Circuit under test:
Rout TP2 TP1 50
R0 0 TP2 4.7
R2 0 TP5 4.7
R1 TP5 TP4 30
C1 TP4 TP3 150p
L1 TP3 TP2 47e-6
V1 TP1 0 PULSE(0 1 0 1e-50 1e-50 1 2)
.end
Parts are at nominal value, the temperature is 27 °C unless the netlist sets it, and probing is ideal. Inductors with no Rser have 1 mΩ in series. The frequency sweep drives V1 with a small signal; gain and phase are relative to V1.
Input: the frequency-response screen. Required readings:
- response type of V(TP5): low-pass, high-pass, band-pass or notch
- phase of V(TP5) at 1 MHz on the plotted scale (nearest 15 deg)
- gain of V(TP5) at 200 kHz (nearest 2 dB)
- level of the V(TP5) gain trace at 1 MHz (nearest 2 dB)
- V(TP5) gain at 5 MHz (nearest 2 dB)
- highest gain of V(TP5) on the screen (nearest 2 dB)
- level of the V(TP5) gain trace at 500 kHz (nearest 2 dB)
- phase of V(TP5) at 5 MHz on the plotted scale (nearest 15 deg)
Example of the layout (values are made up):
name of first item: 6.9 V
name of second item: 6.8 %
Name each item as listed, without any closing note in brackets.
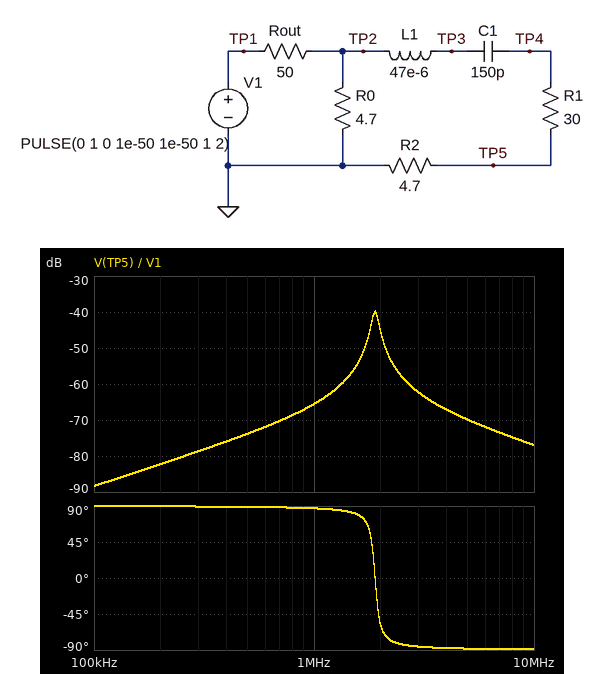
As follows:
response type of V(TP5): low-pass, high-pass, band-pass or notch: band-pass
phase of V(TP5) at 1 MHz on the plotted scale: 90 deg
gain of V(TP5) at 200 kHz: -82 dB
level of the V(TP5) gain trace at 1 MHz: -66 dB
V(TP5) gain at 5 MHz: -70 dB
highest gain of V(TP5) on the screen: -40 dB
level of the V(TP5) gain trace at 500 kHz: -74 dB
phase of V(TP5) at 5 MHz on the plotted scale: -90 deg
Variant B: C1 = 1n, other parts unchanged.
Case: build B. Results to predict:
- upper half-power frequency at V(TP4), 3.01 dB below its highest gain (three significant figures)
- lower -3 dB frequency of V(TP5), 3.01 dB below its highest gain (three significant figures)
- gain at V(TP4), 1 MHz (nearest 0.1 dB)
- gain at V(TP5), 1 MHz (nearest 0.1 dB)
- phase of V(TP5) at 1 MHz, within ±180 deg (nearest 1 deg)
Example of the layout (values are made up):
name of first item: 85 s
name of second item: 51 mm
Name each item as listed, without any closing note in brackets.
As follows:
upper half-power frequency at V(TP4), 3.01 dB below its highest gain: 803 kHz
lower -3 dB frequency of V(TP5), 3.01 dB below its highest gain: 671 kHz
gain at V(TP4), 1 MHz: -33.5 dB
gain at V(TP5), 1 MHz: -50.9 dB
phase of V(TP5) at 1 MHz, within ±180 deg: -74 deg
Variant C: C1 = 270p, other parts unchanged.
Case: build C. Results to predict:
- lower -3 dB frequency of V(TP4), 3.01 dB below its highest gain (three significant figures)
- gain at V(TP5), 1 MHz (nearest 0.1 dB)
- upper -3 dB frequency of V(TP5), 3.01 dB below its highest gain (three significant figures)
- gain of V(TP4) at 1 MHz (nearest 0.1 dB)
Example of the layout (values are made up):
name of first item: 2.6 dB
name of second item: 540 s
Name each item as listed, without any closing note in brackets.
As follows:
lower -3 dB frequency of V(TP4), 3.01 dB below its highest gain: 1.35 MHz
gain at V(TP5), 1 MHz: -57.3 dB
upper -3 dB frequency of V(TP5), 3.01 dB below its highest gain: 1.48 MHz
gain of V(TP4) at 1 MHz: -40.0 dB
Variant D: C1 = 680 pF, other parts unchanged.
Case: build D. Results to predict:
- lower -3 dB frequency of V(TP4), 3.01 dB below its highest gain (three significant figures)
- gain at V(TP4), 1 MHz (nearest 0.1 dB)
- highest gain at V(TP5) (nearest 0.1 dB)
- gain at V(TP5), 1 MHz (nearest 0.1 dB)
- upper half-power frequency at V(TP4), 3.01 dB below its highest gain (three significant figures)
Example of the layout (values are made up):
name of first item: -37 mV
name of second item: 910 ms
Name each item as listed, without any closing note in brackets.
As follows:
lower -3 dB frequency of V(TP4), 3.01 dB below its highest gain: 827 kHz
gain at V(TP4), 1 MHz: -27.7 dB
highest gain at V(TP5): -39.7 dB
gain at V(TP5), 1 MHz: -45.1 dB
upper half-power frequency at V(TP4), 3.01 dB below its highest gain: 959 kHz
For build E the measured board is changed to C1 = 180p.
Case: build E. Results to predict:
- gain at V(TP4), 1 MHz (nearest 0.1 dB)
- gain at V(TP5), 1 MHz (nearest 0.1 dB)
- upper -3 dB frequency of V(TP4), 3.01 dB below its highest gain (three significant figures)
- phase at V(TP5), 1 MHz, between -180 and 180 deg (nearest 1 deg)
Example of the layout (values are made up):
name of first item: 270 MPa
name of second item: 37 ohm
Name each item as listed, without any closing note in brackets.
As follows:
gain at V(TP4), 1 MHz: -45.9 dB
gain at V(TP5), 1 MHz: -63.3 dB
upper -3 dB frequency of V(TP4), 3.01 dB below its highest gain: 1.80 MHz
phase at V(TP5), 1 MHz, between -180 and 180 deg: 86 deg
